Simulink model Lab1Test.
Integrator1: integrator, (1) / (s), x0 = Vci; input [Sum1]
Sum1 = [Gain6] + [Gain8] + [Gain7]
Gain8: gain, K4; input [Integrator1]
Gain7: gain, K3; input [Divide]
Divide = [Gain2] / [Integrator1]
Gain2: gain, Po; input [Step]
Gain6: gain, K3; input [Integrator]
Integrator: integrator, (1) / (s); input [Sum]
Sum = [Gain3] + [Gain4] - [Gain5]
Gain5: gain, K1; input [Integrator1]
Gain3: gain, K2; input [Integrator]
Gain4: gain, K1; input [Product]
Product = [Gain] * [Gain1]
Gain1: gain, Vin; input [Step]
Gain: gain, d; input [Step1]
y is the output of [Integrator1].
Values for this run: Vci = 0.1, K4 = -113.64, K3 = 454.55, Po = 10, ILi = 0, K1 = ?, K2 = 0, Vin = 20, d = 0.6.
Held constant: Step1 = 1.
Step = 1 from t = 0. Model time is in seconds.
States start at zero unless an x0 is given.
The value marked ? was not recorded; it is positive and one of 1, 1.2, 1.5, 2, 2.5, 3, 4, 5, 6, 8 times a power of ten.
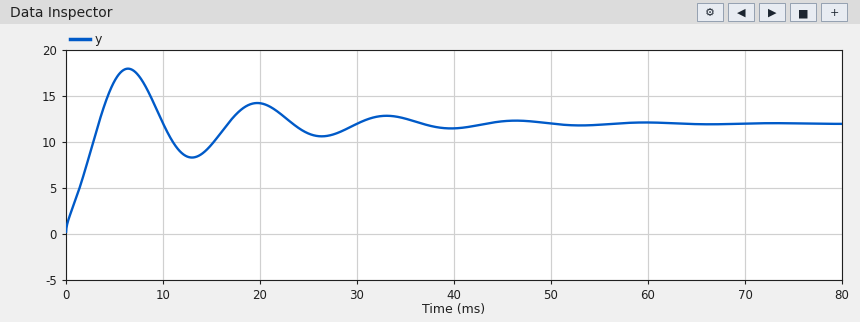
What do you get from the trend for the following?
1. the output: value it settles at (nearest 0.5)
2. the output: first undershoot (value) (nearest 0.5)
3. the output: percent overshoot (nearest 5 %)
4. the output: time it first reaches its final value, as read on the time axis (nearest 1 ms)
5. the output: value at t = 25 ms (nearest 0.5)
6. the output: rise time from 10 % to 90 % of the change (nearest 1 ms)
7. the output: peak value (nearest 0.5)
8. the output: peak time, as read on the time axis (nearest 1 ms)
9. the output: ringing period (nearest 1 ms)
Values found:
12.0
8.5
50 %
3 ms
11.0
3 ms
18.0
6 ms
13 ms
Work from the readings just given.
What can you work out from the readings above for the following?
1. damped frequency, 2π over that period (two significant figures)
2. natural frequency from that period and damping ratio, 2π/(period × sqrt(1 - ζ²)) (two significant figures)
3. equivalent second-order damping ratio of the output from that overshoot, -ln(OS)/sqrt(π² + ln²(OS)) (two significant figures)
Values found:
0.48 rad/ms
0.50 rad/ms
0.22
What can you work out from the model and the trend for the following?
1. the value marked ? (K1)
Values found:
500
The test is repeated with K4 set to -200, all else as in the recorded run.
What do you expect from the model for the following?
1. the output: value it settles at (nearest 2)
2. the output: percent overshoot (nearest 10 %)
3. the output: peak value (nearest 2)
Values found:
12
40 %
16
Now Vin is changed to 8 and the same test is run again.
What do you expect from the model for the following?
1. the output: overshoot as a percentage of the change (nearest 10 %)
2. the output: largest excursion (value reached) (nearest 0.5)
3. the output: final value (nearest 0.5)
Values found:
40 %
6.5
5.0
